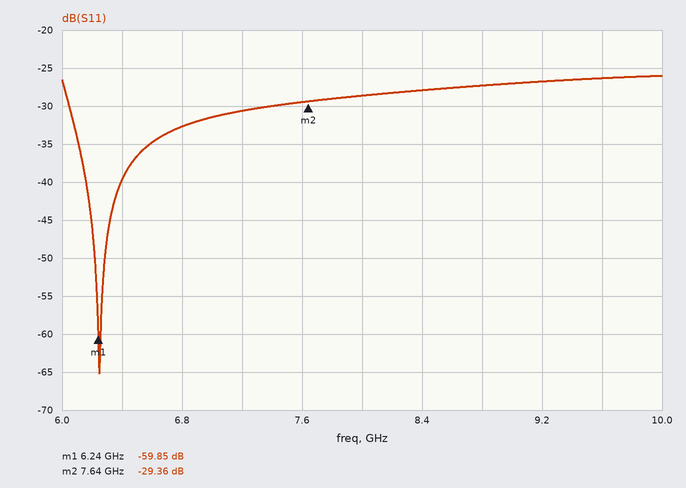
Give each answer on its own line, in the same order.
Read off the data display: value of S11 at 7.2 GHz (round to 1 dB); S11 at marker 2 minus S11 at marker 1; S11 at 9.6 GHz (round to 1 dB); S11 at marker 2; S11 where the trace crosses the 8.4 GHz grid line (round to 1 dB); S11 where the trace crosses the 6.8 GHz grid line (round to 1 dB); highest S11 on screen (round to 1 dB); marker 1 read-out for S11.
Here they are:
-31 dB
30.49 dB
-26 dB
-29.36 dB
-28 dB
-33 dB
-26 dB
-59.85 dB
